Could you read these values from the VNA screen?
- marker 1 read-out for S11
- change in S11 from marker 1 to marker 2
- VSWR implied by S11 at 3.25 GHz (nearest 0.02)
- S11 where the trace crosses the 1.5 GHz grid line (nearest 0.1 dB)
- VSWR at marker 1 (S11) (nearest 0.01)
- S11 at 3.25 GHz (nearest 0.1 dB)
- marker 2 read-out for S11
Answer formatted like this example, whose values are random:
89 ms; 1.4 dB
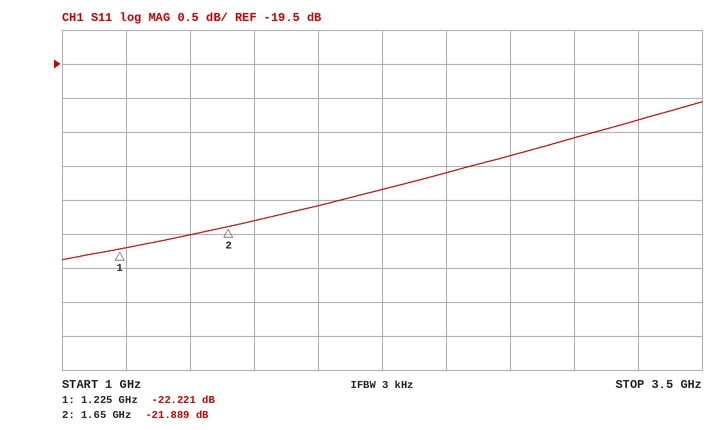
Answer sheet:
-22.221 dB; 0.332 dB; 1.22; -22.0 dB; 1.17; -20.3 dB; -21.889 dB
